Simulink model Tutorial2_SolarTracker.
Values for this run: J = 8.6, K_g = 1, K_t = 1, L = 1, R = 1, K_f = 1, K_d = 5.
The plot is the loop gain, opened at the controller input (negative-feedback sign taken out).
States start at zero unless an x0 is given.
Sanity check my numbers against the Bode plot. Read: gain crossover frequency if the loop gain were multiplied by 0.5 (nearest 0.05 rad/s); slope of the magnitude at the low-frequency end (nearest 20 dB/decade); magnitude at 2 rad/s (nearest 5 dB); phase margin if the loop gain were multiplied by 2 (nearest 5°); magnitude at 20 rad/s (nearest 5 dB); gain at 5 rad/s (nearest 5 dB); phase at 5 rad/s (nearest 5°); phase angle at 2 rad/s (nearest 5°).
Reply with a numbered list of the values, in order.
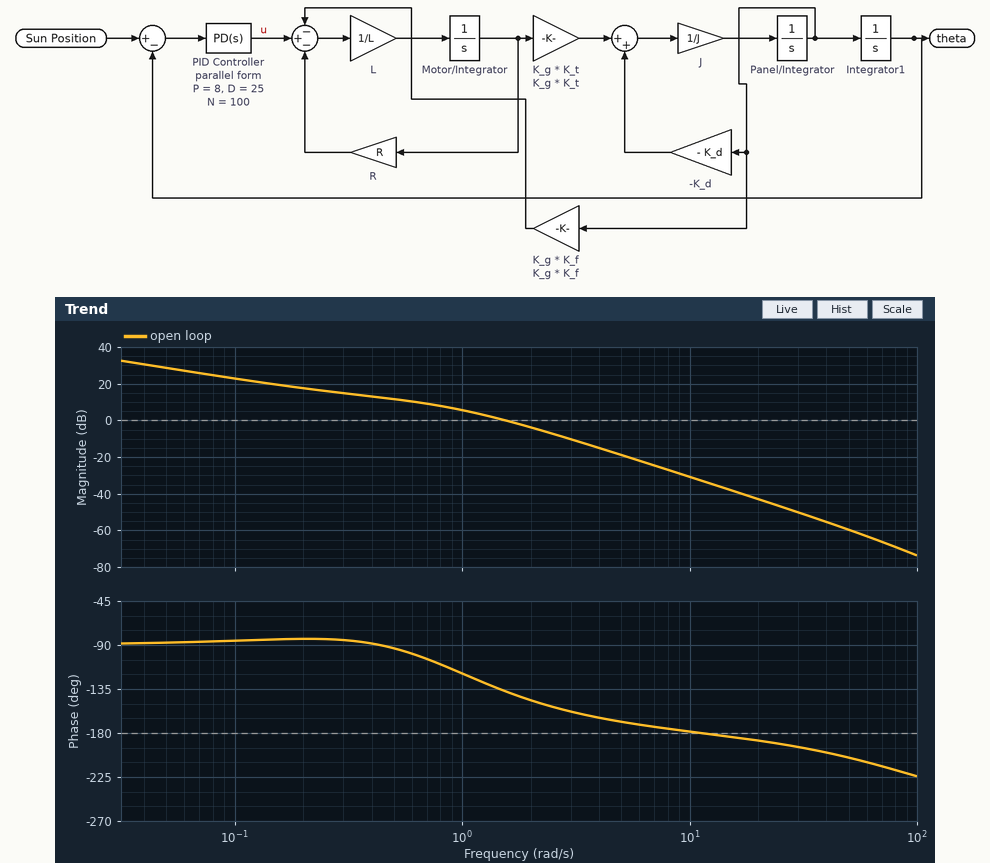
1. 0.95 rad/s
2. -20 dB/decade
3. -5 dB
4. 30°
5. -45 dB
6. -20 dB
7. -170°
8. -145°
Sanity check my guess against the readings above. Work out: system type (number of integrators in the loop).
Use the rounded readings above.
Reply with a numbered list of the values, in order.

1. 1
